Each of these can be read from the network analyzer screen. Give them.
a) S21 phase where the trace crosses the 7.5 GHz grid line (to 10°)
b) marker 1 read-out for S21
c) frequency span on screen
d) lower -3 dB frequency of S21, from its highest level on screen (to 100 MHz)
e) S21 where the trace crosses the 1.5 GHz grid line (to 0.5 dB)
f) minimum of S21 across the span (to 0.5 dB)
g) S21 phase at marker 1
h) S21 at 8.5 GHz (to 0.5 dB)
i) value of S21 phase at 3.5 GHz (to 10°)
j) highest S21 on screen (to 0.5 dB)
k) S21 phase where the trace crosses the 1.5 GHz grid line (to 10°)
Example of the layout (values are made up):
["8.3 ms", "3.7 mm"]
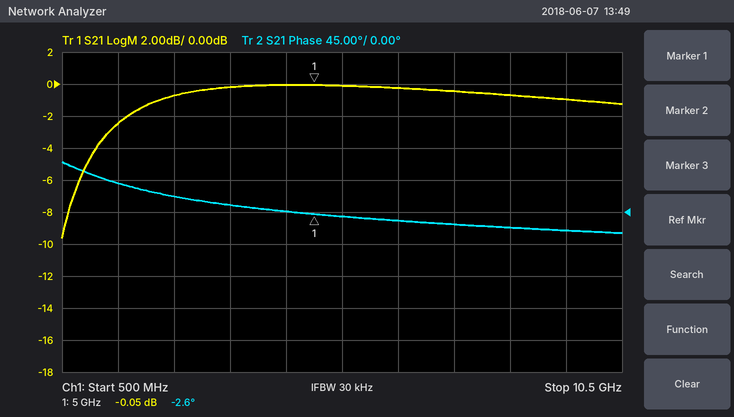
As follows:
["-20°", "-0.05 dB", "10 GHz", "1.3 GHz", "-2.5 dB", "-9.5 dB", "-2.6°", "-0.5 dB", "10°", "0.0 dB", "40°"]
